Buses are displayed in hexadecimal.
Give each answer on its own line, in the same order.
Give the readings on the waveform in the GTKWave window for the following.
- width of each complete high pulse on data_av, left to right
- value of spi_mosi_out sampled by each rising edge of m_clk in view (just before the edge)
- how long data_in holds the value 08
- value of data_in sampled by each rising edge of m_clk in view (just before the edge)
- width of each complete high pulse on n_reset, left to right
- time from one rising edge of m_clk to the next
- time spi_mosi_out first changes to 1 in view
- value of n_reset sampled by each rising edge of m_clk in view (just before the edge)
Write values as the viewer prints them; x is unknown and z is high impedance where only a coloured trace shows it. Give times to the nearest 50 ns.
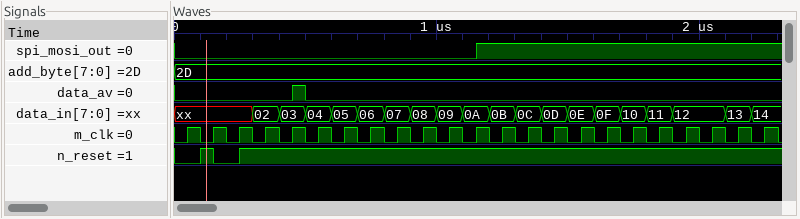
50 ns
0 0 0 0 0 0 0 0 0 0 0 0 1 1 1 1 1 1 1 1 1 1 1
100 ns
xx, xx, xx, 02, 03, 04, 05, 06, 07, 08, 09, 0A, 0B, 0C, 0D, 0E, 0F, 10, 11, 12, 12, 13, 14
50 ns
100 ns
1150 ns
0 1 0 1 1 1 1 1 1 1 1 1 1 1 1 1 1 1 1 1 1 1 1
